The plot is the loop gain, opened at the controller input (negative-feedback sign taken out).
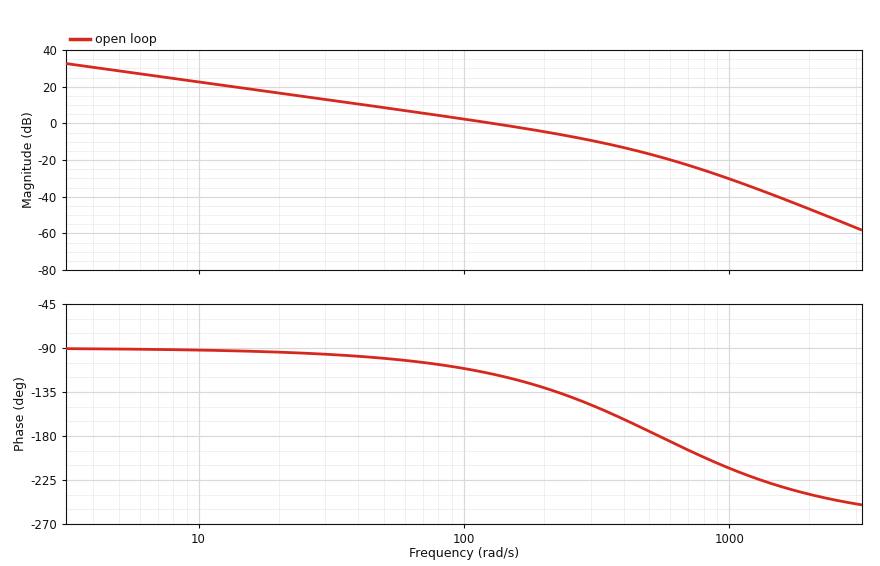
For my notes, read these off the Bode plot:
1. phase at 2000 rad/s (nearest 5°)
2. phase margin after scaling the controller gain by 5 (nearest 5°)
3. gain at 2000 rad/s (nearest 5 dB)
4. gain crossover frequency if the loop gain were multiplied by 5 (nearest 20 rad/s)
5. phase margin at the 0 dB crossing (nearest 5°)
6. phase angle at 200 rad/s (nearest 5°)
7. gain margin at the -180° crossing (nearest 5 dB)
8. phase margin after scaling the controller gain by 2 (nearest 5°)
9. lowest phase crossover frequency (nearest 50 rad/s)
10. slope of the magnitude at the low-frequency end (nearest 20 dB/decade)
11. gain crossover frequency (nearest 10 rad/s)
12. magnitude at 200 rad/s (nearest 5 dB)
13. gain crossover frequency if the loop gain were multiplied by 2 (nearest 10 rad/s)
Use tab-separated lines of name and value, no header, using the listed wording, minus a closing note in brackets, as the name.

phase at 2000 rad/s	-240°
phase margin after scaling the controller gain by 5	15°
gain at 2000 rad/s	-45 dB
gain crossover frequency if the loop gain were multiplied by 5	420 rad/s
phase margin at the 0 dB crossing	65°
phase angle at 200 rad/s	-130°
gain margin at the -180° crossing	20 dB
phase margin after scaling the controller gain by 2	45°
lowest phase crossover frequency	550 rad/s
slope of the magnitude at the low-frequency end	-20 dB/decade
gain crossover frequency	130 rad/s
magnitude at 200 rad/s	-5 dB
gain crossover frequency if the loop gain were multiplied by 2	230 rad/s
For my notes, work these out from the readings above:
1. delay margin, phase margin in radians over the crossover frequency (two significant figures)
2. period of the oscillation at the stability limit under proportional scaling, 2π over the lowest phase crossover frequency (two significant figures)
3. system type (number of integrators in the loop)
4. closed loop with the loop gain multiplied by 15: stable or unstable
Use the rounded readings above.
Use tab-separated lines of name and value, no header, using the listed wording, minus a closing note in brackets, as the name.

delay margin, phase margin in radians over the crossover frequency	0.0087 s
period of the oscillation at the stability limit under proportional scaling, 2π over the lowest phase crossover frequency	0.011 s
system type	1
closed loop with the loop gain multiplied by 15: stable or unstable	unstable
